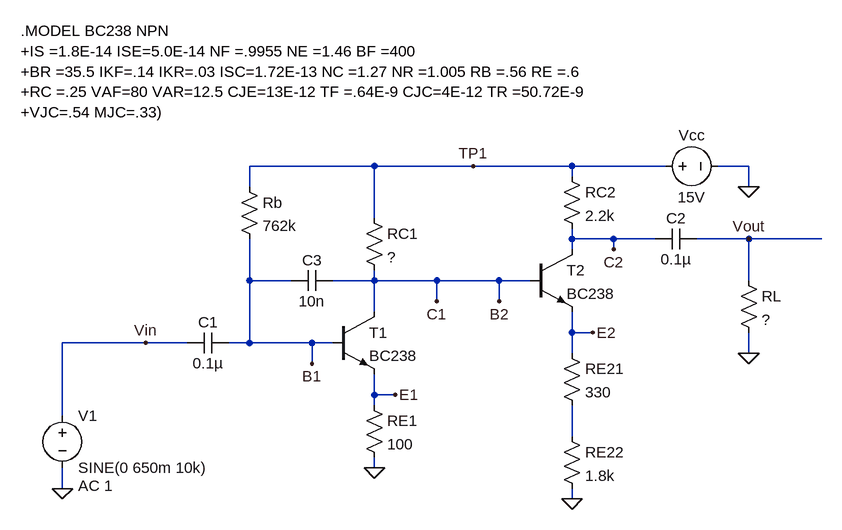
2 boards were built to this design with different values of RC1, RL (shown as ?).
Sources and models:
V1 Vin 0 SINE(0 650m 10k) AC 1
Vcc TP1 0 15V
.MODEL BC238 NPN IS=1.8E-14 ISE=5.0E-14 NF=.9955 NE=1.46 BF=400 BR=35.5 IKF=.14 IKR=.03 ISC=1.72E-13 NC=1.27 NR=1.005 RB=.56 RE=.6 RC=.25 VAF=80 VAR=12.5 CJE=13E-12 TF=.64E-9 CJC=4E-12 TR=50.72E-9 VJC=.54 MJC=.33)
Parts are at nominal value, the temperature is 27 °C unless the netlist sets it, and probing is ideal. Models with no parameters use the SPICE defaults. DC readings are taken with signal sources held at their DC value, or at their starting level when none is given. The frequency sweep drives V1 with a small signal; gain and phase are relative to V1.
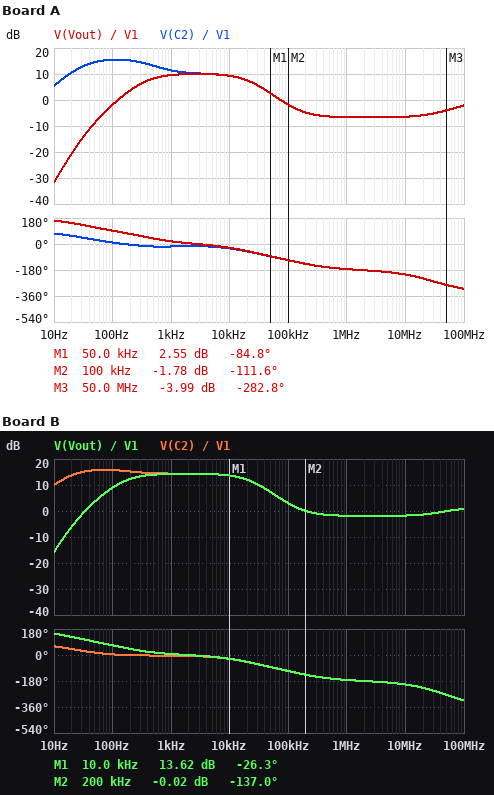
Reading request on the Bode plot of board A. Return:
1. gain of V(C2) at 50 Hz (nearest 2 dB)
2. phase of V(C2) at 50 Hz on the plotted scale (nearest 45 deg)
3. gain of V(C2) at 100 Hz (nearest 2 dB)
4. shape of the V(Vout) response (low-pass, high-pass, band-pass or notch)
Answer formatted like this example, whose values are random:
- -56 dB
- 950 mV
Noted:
- 14 dB
- 45 deg
- 16 dB
- band-pass
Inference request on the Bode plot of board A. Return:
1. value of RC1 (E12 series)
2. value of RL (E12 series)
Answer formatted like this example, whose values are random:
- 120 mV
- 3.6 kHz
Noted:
- 2.7 kΩ
- 2.2 kΩ
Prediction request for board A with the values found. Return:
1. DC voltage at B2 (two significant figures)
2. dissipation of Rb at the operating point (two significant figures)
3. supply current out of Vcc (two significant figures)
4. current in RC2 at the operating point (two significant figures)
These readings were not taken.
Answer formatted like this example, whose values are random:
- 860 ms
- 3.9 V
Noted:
- 810 mV
- 250 µW
- 5.4 mA
- 110 µA
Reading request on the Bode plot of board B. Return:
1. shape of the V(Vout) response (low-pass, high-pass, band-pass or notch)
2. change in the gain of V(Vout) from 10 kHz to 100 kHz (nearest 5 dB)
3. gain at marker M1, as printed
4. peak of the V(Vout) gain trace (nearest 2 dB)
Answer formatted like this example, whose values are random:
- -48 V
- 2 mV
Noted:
- band-pass
- -10 dB
- 13.62 dB
- 14 dB
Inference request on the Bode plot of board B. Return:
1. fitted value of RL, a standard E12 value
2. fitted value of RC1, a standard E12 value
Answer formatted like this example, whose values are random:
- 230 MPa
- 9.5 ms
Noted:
- 8.2 kΩ
- 2.2 kΩ
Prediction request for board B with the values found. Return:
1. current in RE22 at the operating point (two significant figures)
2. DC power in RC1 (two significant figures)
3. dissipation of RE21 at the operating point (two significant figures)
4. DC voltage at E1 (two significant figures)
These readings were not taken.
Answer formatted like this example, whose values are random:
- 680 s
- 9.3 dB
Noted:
- 1.1 mA
- 65 mW
- 430 µW
- 540 mV
